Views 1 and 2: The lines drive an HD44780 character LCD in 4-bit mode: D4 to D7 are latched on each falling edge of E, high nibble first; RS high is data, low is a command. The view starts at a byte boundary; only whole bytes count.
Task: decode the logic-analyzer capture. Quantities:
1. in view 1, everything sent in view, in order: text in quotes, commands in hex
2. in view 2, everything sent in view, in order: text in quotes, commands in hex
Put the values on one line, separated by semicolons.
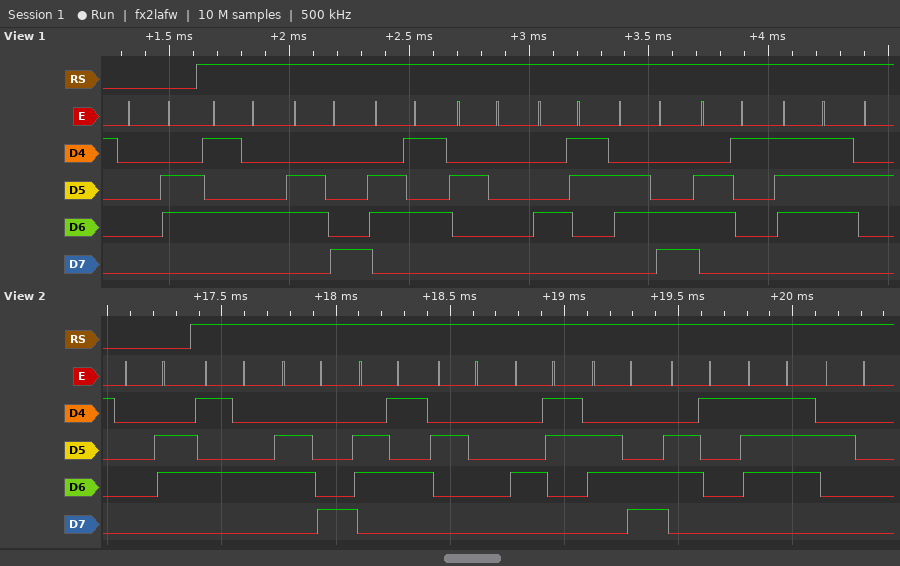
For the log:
0x06 "The Claw"; 0x06 "The Claw "
